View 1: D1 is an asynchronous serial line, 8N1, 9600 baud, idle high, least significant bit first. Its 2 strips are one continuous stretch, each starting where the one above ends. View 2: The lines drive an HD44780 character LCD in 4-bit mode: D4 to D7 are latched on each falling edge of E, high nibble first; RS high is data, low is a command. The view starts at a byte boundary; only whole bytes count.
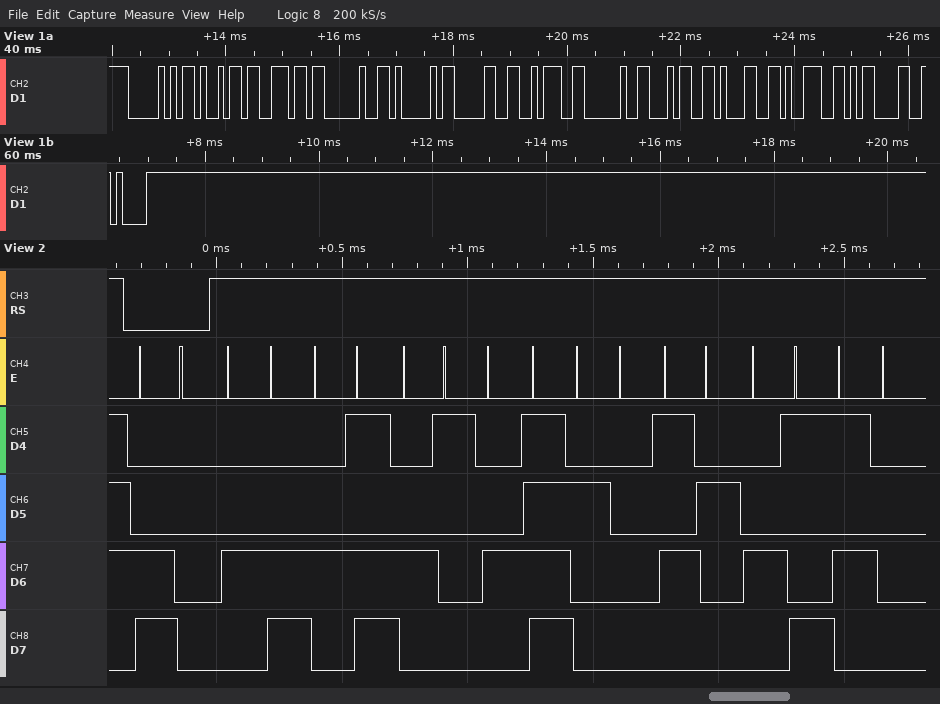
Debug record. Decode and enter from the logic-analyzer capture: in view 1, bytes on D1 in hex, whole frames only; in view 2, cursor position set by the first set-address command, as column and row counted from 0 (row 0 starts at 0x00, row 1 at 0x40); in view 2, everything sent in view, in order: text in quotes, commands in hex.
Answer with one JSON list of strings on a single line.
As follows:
["0x50 0x69 0x6E 0x20 0x41 0x30 0x3A 0x20 0x34 0x31 0x39 0x0D 0x0A", "column 0, row 1", "0xC0 \"LMAO RIP\""]
